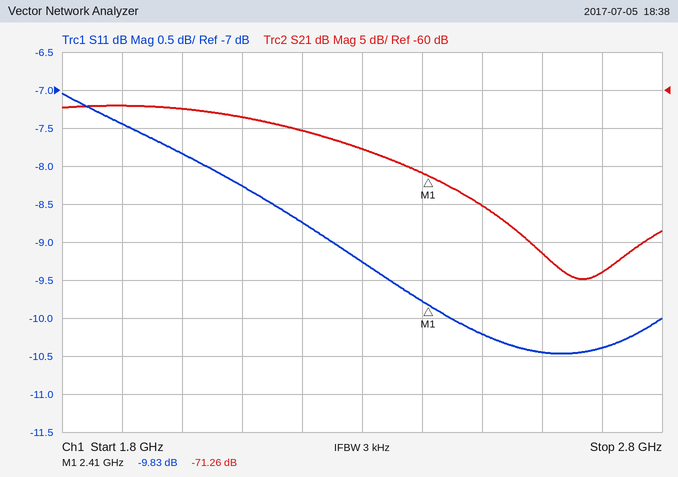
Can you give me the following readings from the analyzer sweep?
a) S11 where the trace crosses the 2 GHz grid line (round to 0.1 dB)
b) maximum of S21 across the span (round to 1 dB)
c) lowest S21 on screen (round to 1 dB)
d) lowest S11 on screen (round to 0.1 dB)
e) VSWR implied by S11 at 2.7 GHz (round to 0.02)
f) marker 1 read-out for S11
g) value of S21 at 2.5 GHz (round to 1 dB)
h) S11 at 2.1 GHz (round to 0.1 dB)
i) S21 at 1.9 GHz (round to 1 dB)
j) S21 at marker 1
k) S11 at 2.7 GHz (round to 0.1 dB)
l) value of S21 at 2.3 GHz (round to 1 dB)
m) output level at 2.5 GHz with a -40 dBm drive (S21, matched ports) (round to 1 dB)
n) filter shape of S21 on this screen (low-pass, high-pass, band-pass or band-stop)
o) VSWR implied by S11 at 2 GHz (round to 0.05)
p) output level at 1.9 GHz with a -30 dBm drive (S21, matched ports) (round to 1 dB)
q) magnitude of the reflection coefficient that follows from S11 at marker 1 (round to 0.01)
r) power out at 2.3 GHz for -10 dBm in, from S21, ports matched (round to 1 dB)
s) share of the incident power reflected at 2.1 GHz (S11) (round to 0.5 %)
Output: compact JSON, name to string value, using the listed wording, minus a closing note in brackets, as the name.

{"S11 where the trace crosses the 2 GHz grid line": "-7.8 dB", "maximum of S21 across the span": "-62 dB", "lowest S21 on screen": "-85 dB", "lowest S11 on screen": "-10.5 dB", "VSWR implied by S11 at 2.7 GHz": "1.86", "marker 1 read-out for S11": "-9.83 dB", "value of S21 at 2.5 GHz": "-75 dB", "S11 at 2.1 GHz": "-8.3 dB", "S21 at 1.9 GHz": "-62 dB", "S21 at marker 1": "-71.26 dB", "S11 at 2.7 GHz": "-10.4 dB", "value of S21 at 2.3 GHz": "-68 dB", "output level at 2.5 GHz with a -40 dBm drive (S21, matched ports)": "-115 dBm", "filter shape of S21 on this screen": "low-pass", "VSWR implied by S11 at 2 GHz": "2.35", "output level at 1.9 GHz with a -30 dBm drive (S21, matched ports)": "-92 dBm", "magnitude of the reflection coefficient that follows from S11 at marker 1": "0.32", "power out at 2.3 GHz for -10 dBm in, from S21, ports matched": "-78 dBm", "share of the incident power reflected at 2.1 GHz (S11)": "15.0 %"}
